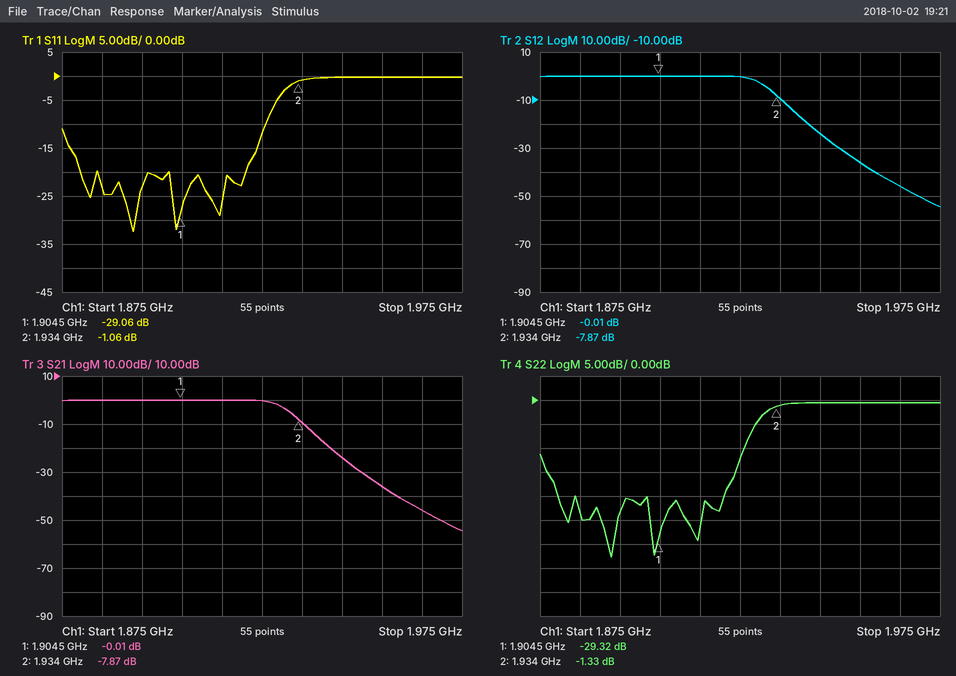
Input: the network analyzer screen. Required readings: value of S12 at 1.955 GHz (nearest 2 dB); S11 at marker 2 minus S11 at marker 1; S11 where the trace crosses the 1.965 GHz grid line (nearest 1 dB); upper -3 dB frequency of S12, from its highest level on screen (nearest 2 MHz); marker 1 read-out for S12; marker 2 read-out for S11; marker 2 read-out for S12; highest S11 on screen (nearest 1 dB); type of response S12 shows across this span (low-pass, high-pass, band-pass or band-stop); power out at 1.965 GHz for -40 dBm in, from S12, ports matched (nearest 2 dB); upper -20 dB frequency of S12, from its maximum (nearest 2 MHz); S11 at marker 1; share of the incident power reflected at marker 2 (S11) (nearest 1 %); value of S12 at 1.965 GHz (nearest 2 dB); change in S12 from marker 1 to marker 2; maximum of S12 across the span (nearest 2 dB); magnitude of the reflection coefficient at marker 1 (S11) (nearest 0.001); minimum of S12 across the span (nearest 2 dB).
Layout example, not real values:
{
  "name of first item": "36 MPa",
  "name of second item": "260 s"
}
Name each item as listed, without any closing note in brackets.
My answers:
{
  "value of S12 at 1.955 GHz": "-36 dB",
  "S11 at marker 2 minus S11 at marker 1": "28.00 dB",
  "S11 where the trace crosses the 1.965 GHz grid line": "0 dB",
  "upper -3 dB frequency of S12, from its highest level on screen": "1.930 GHz",
  "marker 1 read-out for S12": "-0.01 dB",
  "marker 2 read-out for S11": "-1.06 dB",
  "marker 2 read-out for S12": "-7.87 dB",
  "highest S11 on screen": "0 dB",
  "type of response S12 shows across this span": "low-pass",
  "power out at 1.965 GHz for -40 dBm in, from S12, ports matched": "-86 dBm",
  "upper -20 dB frequency of S12, from its maximum": "1.942 GHz",
  "S11 at marker 1": "-29.06 dB",
  "share of the incident power reflected at marker 2 (S11)": "78 %",
  "value of S12 at 1.965 GHz": "-46 dB",
  "change in S12 from marker 1 to marker 2": "-7.86 dB",
  "maximum of S12 across the span": "0 dB",
  "magnitude of the reflection coefficient at marker 1 (S11)": "0.035",
  "minimum of S12 across the span": "-54 dB"
}
